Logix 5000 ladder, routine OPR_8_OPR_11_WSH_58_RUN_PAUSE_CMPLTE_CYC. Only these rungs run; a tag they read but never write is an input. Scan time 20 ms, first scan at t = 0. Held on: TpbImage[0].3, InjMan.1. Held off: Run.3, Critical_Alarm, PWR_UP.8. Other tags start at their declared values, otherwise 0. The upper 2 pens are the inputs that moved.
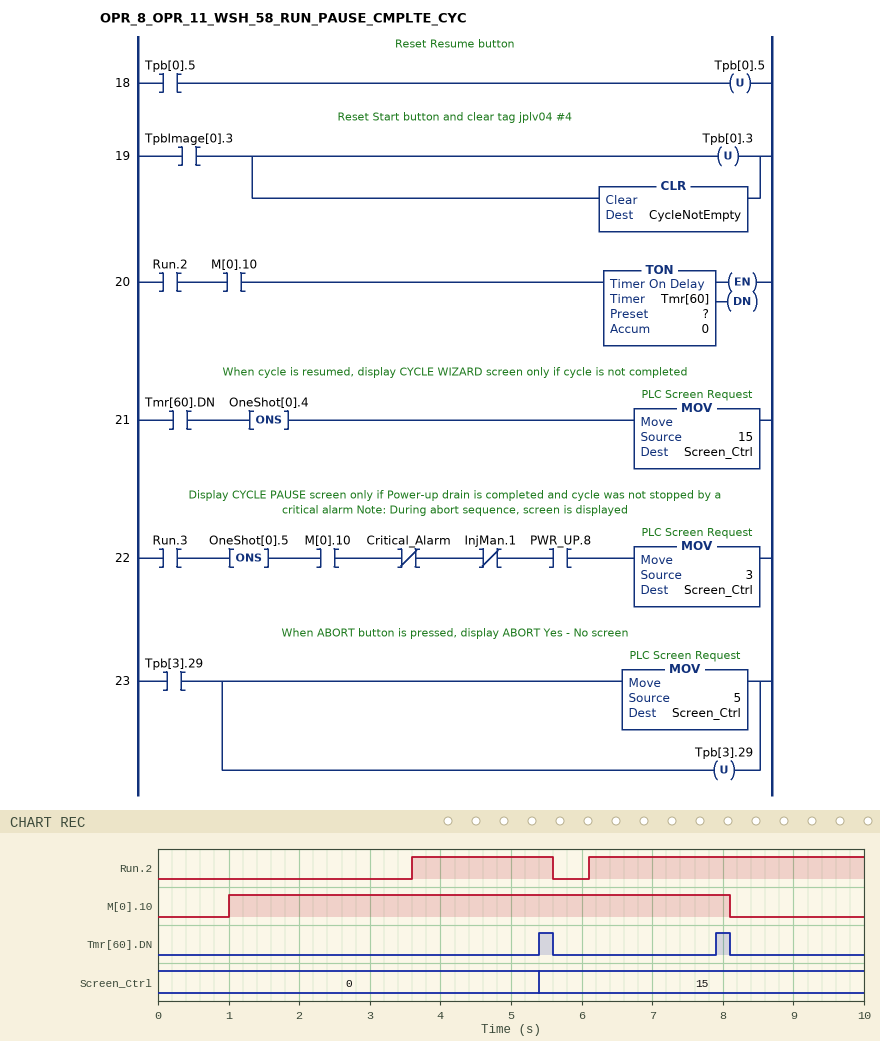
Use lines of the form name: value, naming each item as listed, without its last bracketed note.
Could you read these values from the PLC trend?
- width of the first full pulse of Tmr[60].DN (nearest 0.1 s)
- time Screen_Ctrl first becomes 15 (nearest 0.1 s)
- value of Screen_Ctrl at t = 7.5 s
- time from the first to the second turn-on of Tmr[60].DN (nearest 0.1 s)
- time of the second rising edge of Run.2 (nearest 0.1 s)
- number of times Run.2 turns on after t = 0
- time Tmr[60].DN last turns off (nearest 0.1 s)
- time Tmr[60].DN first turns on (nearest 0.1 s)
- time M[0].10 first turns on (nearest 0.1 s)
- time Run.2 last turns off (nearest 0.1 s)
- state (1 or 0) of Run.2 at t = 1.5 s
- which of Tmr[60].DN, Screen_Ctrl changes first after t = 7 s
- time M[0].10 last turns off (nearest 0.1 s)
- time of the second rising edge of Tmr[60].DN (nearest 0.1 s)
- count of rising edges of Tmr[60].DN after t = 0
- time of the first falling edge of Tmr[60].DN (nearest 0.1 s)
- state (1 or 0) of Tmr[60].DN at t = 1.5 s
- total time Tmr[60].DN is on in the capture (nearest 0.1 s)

width of the first full pulse of Tmr[60].DN: 0.2 s
time Screen_Ctrl first becomes 15: 5.4 s
value of Screen_Ctrl at t = 7.5 s: 15
time from the first to the second turn-on of Tmr[60].DN: 2.5 s
time of the second rising edge of Run.2: 6.1 s
number of times Run.2 turns on after t = 0: 2
time Tmr[60].DN last turns off: 8.1 s
time Tmr[60].DN first turns on: 5.4 s
time M[0].10 first turns on: 1.0 s
time Run.2 last turns off: 5.6 s
state (1 or 0) of Run.2 at t = 1.5 s: 0
which of Tmr[60].DN, Screen_Ctrl changes first after t = 7 s: Tmr[60].DN
time M[0].10 last turns off: 8.1 s
time of the second rising edge of Tmr[60].DN: 7.9 s
count of rising edges of Tmr[60].DN after t = 0: 2
time of the first falling edge of Tmr[60].DN: 5.6 s
state (1 or 0) of Tmr[60].DN at t = 1.5 s: 0
total time Tmr[60].DN is on in the capture: 0.4 s
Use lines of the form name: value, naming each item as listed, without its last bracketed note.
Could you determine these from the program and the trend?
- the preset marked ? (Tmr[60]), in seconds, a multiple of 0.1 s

the preset marked ? (Tmr[60]), in seconds, a multiple of 0.1 s: 1.8 s
